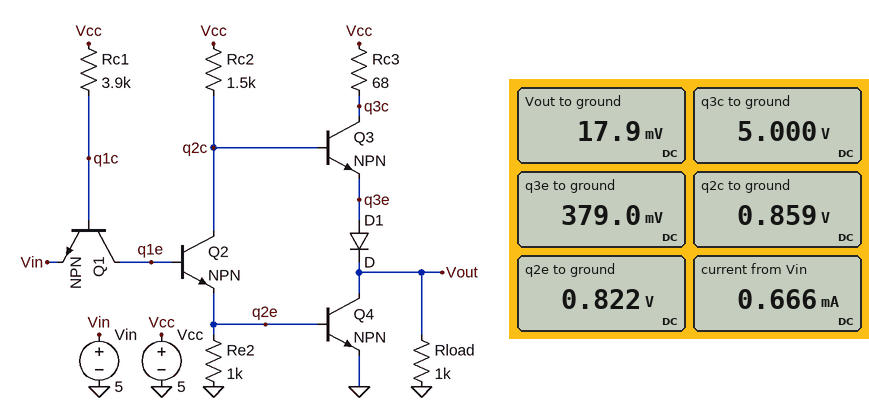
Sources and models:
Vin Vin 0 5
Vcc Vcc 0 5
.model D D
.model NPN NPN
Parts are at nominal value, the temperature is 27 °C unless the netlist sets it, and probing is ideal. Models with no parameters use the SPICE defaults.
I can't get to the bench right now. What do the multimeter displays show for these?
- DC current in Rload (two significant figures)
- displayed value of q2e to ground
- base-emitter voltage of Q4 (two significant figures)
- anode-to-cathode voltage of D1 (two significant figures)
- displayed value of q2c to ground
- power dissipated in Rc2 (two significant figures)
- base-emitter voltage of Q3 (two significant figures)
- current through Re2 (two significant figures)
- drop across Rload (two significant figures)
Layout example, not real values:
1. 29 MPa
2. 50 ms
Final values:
1. 18 µA
2. 0.822 V
3. 820 mV
4. 360 mV
5. 0.859 V
6. 11 mW
7. 480 mV
8. 820 µA
9. 18 mV
